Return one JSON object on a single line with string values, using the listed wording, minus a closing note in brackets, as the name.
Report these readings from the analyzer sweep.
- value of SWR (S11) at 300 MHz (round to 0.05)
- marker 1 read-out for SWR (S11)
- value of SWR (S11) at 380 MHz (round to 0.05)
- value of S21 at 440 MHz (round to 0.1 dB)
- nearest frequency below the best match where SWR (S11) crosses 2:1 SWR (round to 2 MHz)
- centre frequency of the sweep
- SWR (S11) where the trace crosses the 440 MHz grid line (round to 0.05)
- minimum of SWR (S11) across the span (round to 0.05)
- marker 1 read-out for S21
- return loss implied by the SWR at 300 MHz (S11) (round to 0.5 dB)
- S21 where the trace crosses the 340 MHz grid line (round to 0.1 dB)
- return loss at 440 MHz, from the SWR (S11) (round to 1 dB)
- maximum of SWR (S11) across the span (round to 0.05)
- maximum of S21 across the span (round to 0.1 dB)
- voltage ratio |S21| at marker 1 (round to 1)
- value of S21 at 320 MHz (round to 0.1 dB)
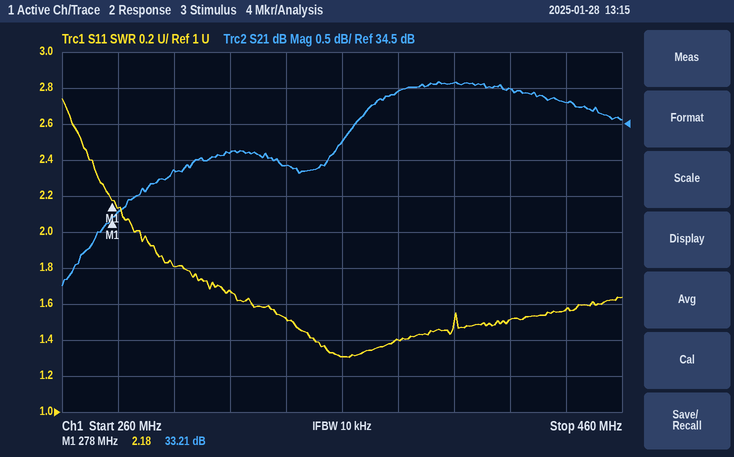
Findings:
{"value of SWR (S11) at 300 MHz": "1.80", "marker 1 read-out for SWR": "2.18", "value of SWR (S11) at 380 MHz": "1.40", "value of S21 at 440 MHz": "34.8 dB", "nearest frequency below the best match where SWR (S11) crosses 2:1 SWR": "288 MHz", "centre frequency of the sweep": "360 MHz", "SWR (S11) where the trace crosses the 440 MHz grid line": "1.55", "minimum of SWR (S11) across the span": "1.30", "marker 1 read-out for S21": "33.21 dB", "return loss implied by the SWR at 300 MHz (S11)": "11.0 dB", "S21 where the trace crosses the 340 MHz grid line": "33.9 dB", "return loss at 440 MHz, from the SWR (S11)": "13 dB", "maximum of SWR (S11) across the span": "2.75", "maximum of S21 across the span": "35.1 dB", "voltage ratio |S21| at marker 1": "46", "value of S21 at 320 MHz": "34.1 dB"}
